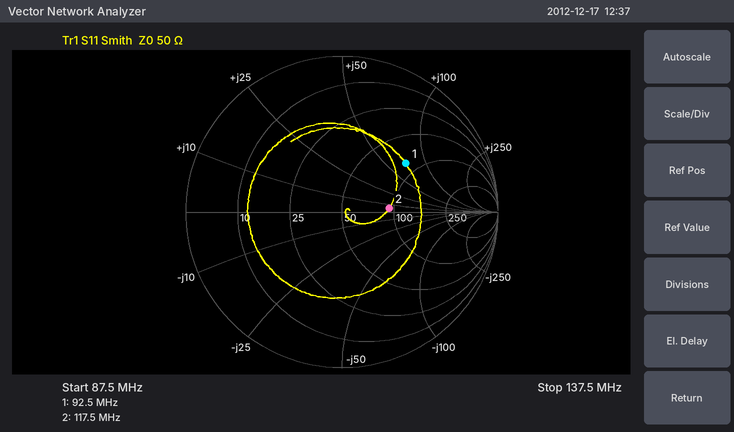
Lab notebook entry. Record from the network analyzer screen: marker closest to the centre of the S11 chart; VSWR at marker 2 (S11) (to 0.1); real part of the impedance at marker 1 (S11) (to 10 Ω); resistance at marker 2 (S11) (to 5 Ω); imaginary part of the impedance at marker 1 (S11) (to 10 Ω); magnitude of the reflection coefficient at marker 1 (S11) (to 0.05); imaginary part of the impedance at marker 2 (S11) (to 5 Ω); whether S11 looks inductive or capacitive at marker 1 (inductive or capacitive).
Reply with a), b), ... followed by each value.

a) marker 2
b) 1.9
c) 80 Ω
d) 95 Ω
e) +70 Ω
f) 0.50
g) +5 Ω
h) inductive
